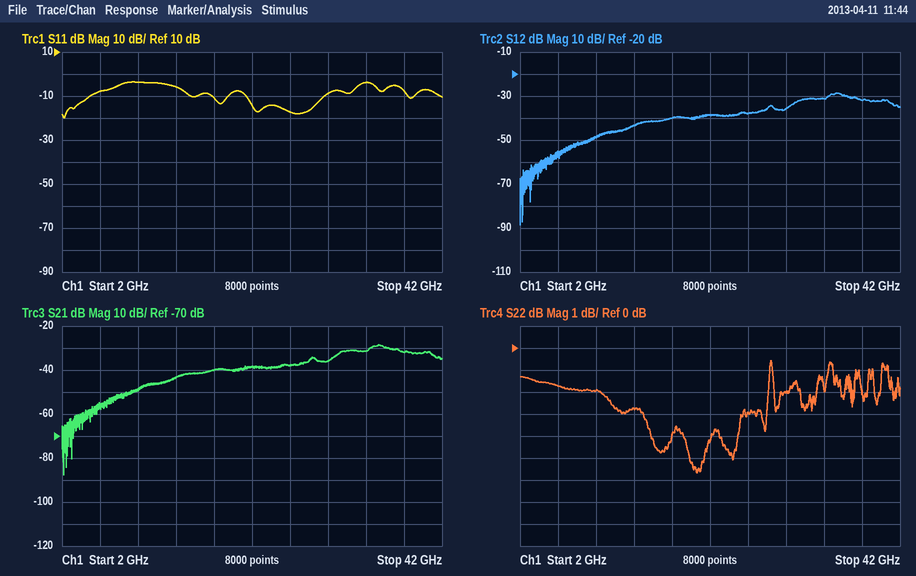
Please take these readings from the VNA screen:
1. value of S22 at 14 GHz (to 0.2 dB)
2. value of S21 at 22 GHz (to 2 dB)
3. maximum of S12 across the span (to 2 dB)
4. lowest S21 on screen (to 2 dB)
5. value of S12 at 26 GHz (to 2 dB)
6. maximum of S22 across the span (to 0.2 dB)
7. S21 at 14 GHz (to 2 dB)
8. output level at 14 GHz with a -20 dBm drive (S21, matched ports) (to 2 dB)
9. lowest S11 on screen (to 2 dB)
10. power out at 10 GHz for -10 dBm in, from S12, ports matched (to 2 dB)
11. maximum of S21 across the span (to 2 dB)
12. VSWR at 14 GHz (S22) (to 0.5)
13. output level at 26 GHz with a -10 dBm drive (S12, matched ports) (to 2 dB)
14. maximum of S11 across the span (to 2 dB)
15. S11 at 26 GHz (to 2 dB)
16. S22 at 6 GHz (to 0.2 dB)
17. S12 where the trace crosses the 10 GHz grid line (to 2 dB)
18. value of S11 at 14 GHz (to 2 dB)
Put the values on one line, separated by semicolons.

-2.8 dB; -38 dB; -28 dB; -88 dB; -38 dB; -0.6 dB; -44 dB; -64 dBm; -20 dB; -58 dBm; -28 dB; 6.5; -48 dBm; -4 dB; -18 dB; -1.8 dB; -48 dB; -6 dB
